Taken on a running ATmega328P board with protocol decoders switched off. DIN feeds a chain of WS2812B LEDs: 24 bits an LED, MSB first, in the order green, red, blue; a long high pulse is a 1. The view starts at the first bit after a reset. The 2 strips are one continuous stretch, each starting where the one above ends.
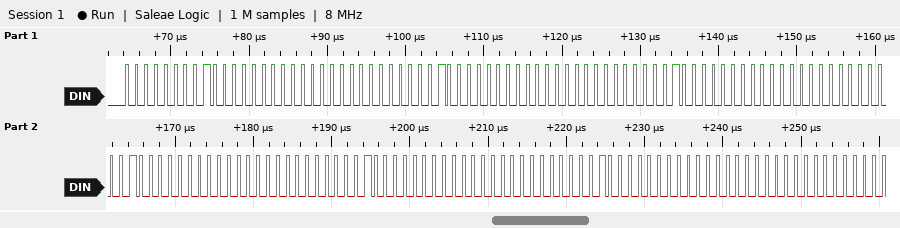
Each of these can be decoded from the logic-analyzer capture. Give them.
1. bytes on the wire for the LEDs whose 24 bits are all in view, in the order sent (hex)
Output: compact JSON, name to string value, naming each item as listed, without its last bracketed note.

{"bytes on the wire for the LEDs whose 24 bits are all in view, in the order sent": "00 80 00 00 80 00 00 80 00 00 80 00 00 80 00 00 80 00"}
